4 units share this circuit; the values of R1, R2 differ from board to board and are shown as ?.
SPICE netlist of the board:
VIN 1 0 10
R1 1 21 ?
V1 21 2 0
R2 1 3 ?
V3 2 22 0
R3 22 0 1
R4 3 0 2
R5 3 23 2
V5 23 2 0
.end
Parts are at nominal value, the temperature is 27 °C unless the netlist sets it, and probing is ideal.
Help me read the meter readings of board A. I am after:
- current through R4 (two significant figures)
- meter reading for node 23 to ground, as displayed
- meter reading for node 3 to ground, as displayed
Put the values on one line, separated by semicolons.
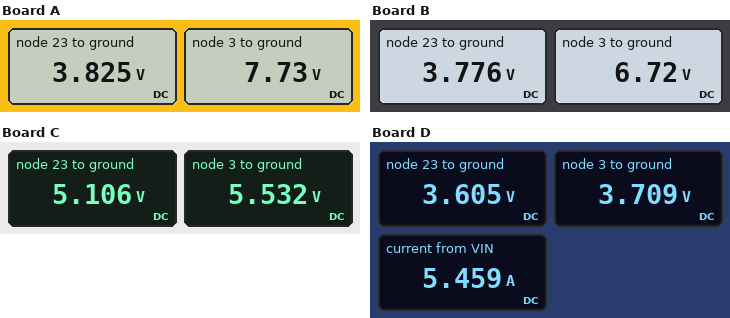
3.9 A; 3.825 V; 7.73 V
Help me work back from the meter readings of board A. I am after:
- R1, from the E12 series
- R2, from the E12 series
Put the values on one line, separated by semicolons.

3.3 Ω; 0.39 Ω
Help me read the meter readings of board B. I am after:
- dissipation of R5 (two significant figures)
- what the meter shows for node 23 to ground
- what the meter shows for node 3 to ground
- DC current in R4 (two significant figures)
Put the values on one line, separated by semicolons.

4.3 W; 3.776 V; 6.72 V; 3.4 A
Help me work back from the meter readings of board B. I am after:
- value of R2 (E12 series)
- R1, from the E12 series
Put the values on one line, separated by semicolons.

0.68 Ω; 2.7 Ω
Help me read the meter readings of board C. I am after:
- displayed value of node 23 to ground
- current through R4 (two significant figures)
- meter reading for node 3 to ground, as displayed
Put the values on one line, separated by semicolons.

5.106 V; 2.8 A; 5.532 V
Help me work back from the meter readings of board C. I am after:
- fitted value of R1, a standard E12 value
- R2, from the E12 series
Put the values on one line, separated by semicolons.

1 Ω; 1.5 Ω
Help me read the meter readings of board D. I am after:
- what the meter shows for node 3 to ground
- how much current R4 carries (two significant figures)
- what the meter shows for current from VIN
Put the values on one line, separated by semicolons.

3.709 V; 1.9 A; 5.459 A
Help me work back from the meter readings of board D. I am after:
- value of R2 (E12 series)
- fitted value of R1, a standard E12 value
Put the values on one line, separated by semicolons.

3.3 Ω; 1.8 Ω
